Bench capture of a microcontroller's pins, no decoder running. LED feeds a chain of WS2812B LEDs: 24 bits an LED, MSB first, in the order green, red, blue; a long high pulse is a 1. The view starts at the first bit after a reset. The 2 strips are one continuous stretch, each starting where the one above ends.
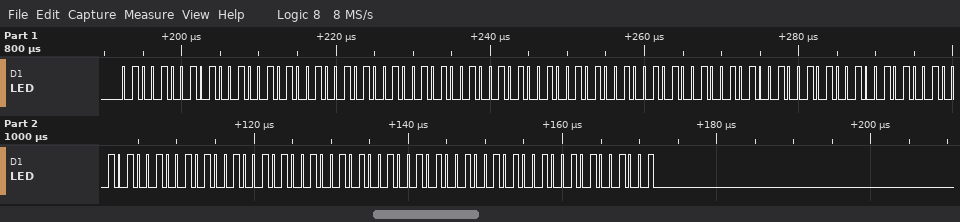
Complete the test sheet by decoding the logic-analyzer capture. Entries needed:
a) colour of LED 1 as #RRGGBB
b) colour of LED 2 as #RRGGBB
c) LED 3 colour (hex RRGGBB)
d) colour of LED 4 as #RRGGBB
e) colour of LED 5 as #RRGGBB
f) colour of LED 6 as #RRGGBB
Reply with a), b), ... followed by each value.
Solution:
a) #494949
b) #494949
c) #494949
d) #494949
e) #494949
f) #494949
